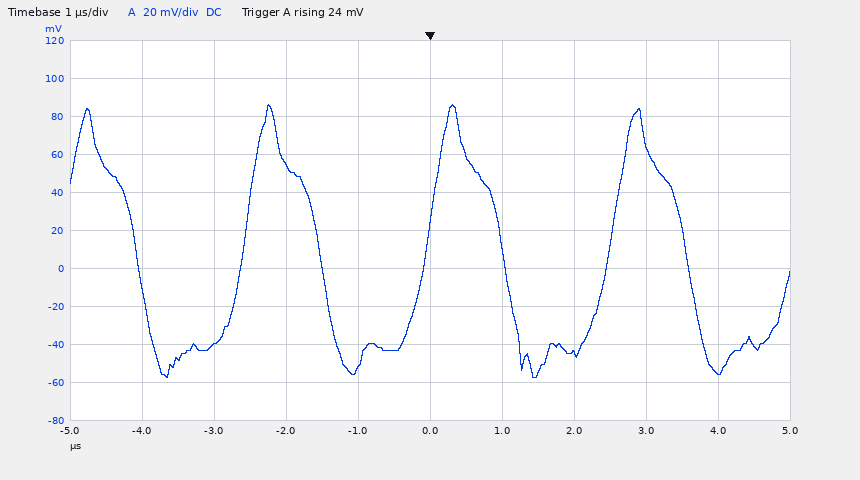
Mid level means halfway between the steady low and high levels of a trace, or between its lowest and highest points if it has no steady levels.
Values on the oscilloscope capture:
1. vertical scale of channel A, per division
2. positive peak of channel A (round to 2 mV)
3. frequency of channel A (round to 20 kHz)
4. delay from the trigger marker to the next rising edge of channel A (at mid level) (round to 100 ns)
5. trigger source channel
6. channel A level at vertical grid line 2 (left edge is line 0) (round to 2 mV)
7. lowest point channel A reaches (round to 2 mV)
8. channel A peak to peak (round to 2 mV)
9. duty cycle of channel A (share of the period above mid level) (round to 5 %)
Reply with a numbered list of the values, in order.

1. 20 mV
2. 86 mV
3. 400 kHz
4. 2.5 µs
5. channel A
6. -40 mV
7. -58 mV
8. 144 mV
9. 40 %
